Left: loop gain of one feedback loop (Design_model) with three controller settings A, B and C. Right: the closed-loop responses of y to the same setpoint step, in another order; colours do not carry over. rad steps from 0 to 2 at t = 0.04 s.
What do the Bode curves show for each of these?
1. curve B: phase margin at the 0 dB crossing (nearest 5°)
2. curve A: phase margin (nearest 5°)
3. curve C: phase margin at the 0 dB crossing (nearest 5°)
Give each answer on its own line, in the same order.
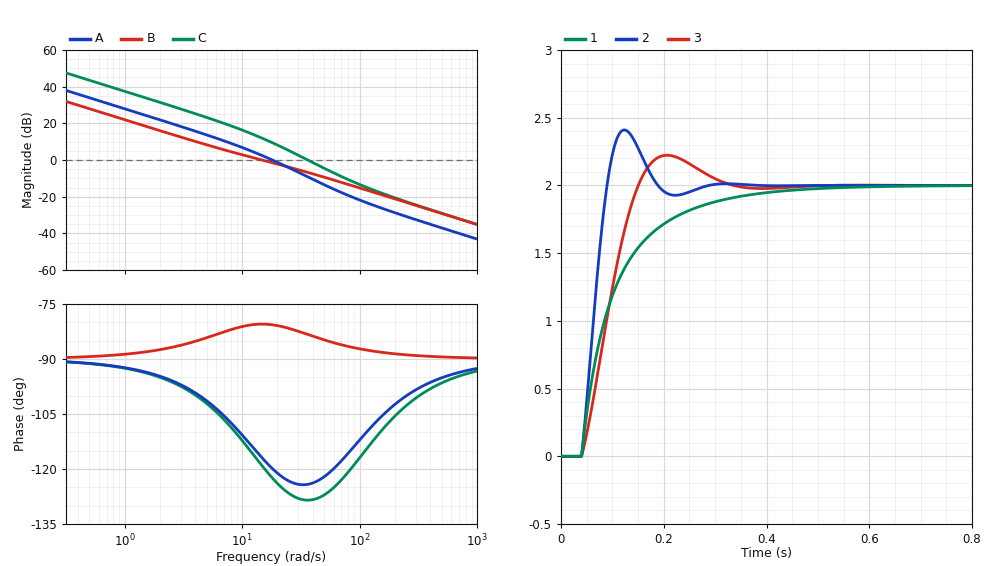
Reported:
100°
60°
50°
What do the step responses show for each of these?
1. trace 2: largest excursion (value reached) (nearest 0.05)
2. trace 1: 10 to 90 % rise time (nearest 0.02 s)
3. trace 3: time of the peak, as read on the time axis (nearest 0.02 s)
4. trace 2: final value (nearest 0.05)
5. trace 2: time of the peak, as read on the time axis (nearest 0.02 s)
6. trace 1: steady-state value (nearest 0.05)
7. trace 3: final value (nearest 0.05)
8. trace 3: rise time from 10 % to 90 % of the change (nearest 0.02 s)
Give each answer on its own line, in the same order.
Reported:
2.40
0.20 s
0.20 s
2.00
0.12 s
2.00
2.00
0.08 s
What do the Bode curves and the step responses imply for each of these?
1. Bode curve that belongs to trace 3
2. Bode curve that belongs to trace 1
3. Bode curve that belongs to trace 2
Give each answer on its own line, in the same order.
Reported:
A
B
C
